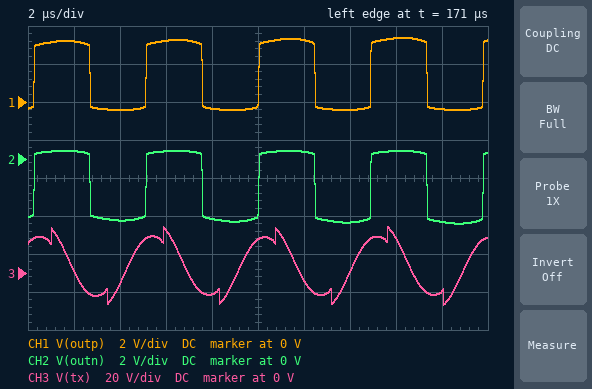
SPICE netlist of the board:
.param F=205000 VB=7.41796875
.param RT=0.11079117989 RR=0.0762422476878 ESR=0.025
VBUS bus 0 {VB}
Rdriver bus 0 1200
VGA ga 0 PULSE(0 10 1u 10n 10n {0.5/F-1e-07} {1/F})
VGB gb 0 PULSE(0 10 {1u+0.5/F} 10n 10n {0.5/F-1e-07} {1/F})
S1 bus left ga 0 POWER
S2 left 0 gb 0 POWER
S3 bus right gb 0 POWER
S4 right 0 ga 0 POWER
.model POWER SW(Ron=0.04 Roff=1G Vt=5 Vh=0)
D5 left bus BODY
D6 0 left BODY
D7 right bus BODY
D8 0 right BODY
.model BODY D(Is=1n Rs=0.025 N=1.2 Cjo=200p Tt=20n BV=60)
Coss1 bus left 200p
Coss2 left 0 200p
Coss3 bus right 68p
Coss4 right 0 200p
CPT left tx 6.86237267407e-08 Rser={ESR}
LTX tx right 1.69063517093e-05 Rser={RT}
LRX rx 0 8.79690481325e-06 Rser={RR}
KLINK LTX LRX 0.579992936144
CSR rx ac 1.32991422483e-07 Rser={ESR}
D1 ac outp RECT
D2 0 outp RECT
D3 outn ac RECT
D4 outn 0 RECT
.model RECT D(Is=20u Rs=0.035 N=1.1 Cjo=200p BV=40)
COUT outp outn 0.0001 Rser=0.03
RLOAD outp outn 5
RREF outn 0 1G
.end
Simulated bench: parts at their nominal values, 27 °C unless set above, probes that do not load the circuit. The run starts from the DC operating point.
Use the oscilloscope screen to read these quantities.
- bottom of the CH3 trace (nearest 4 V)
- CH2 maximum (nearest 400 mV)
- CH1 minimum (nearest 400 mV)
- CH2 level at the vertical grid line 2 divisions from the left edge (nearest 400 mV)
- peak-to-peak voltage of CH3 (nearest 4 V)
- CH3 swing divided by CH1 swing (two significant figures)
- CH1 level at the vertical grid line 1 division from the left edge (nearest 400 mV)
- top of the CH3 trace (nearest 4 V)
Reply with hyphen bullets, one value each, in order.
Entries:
- -16 V
- 400 mV
- -400 mV
- -3.2 V
- 40 V
- 11
- 3.2 V
- 24 V
